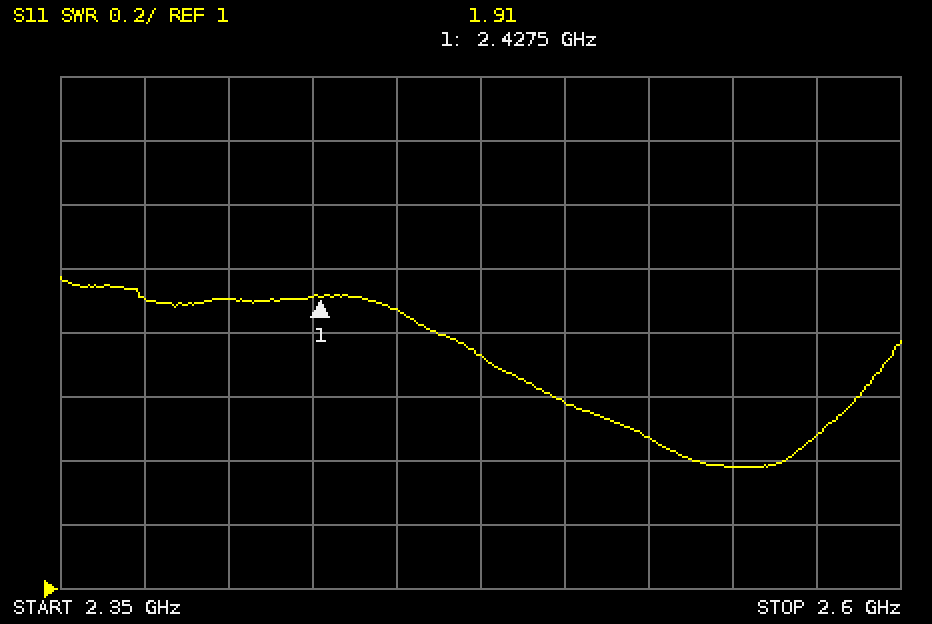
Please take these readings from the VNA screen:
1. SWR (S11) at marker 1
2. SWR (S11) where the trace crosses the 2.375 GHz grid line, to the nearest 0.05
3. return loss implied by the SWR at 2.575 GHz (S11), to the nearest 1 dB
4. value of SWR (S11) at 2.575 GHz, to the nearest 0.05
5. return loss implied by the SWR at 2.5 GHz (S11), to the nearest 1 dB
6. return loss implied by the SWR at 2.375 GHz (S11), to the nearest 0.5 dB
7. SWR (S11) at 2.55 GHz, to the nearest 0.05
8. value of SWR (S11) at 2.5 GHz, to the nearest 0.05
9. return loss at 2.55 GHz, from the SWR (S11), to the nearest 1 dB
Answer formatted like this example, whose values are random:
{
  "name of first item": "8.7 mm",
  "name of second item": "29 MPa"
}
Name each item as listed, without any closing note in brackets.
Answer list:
{
  "SWR (S11) at marker 1": "1.91",
  "SWR (S11) where the trace crosses the 2.375 GHz grid line, to the nearest 0.05": "1.90",
  "return loss implied by the SWR at 2.575 GHz (S11), to the nearest 1 dB": "14 dB",
  "value of SWR (S11) at 2.575 GHz, to the nearest 0.05": "1.50",
  "return loss implied by the SWR at 2.5 GHz (S11), to the nearest 1 dB": "13 dB",
  "return loss implied by the SWR at 2.375 GHz (S11), to the nearest 0.5 dB": "10.0 dB",
  "SWR (S11) at 2.55 GHz, to the nearest 0.05": "1.40",
  "value of SWR (S11) at 2.5 GHz, to the nearest 0.05": "1.60",
  "return loss at 2.55 GHz, from the SWR (S11), to the nearest 1 dB": "16 dB"
}
